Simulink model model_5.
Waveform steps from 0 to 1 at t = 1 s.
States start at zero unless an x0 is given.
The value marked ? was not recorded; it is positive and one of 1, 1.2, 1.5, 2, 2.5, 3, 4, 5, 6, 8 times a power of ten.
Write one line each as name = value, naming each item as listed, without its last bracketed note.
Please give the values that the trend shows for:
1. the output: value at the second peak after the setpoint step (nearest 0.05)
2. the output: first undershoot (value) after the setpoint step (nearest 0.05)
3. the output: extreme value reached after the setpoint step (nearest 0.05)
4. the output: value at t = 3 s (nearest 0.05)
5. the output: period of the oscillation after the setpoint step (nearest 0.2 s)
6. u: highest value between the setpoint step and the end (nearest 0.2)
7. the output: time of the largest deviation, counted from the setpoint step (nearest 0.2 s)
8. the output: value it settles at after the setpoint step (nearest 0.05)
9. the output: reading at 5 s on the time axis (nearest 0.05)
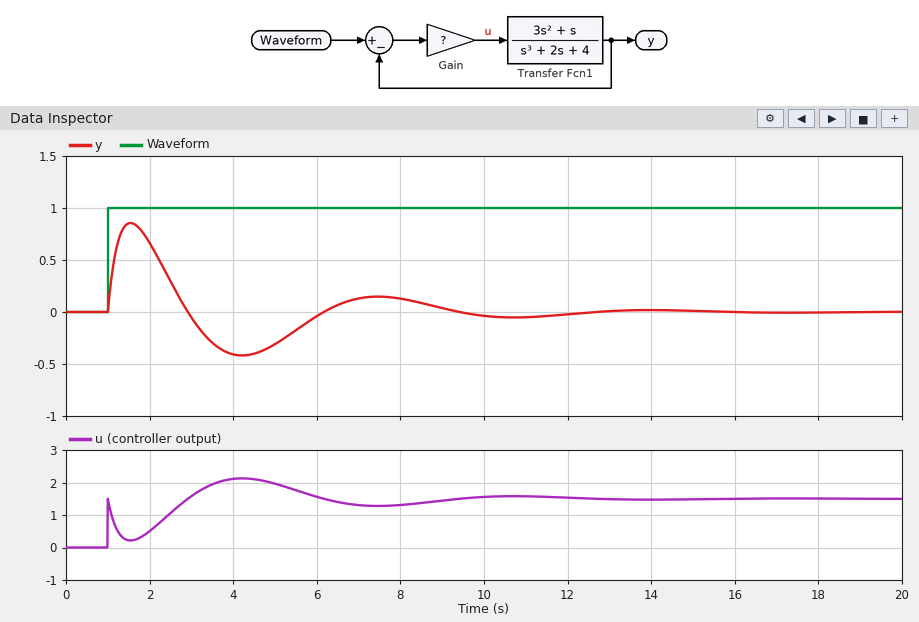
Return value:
the output: value at the second peak after the setpoint step = 0.15
the output: first undershoot (value) after the setpoint step = -0.40
the output: extreme value reached after the setpoint step = 0.85
the output: value at t = 3 s = -0.05
the output: period of the oscillation after the setpoint step = 6.0 s
u: highest value between the setpoint step and the end = 2.2
the output: time of the largest deviation, counted from the setpoint step = 0.6 s
the output: value it settles at after the setpoint step = 0.00
the output: reading at 5 s on the time axis = -0.30
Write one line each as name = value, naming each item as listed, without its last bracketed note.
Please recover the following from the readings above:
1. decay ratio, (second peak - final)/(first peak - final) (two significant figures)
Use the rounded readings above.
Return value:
decay ratio, (second peak - final)/(first peak - final) = 0.18
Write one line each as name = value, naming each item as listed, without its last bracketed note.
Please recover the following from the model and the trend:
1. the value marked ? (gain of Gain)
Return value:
the value marked ? = 1.5
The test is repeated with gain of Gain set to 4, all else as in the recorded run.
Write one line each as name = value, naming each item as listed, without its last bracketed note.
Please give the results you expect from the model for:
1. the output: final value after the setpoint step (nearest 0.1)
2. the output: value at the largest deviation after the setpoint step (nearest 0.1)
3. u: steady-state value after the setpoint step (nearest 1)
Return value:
the output: final value after the setpoint step = 0.0
the output: value at the largest deviation after the setpoint step = 1.0
u: steady-state value after the setpoint step = 4
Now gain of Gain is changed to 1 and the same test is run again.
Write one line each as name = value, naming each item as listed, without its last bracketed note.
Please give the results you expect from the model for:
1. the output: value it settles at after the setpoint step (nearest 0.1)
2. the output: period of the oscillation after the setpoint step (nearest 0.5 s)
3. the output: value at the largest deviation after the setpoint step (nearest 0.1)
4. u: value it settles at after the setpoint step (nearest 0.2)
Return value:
the output: value it settles at after the setpoint step = 0.0
the output: period of the oscillation after the setpoint step = 4.5 s
the output: value at the largest deviation after the setpoint step = 0.8
u: value it settles at after the setpoint step = 1.0
